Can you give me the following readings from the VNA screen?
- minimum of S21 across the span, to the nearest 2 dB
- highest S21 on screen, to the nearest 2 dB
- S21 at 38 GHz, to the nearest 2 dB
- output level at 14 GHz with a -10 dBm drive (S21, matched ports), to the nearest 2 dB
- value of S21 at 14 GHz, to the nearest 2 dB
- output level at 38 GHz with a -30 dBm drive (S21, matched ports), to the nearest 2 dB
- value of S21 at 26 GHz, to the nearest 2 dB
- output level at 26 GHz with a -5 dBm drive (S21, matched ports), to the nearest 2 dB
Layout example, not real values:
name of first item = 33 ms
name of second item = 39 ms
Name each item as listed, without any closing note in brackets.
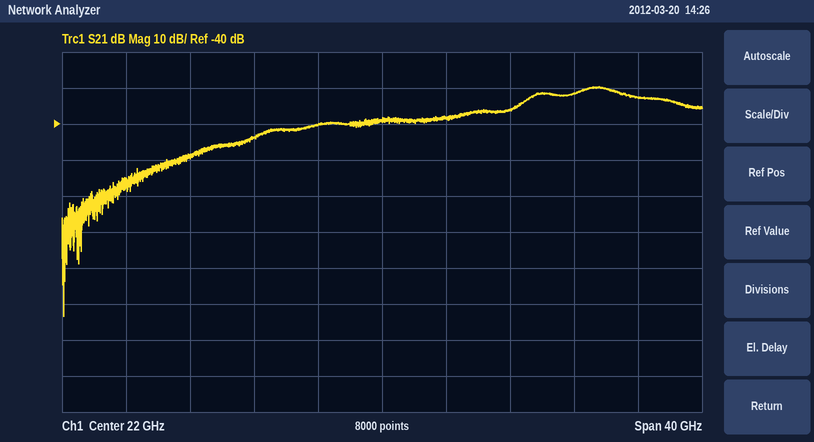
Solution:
minimum of S21 across the span, to the nearest 2 dB = -94 dB
highest S21 on screen, to the nearest 2 dB = -30 dB
S21 at 38 GHz, to the nearest 2 dB = -32 dB
output level at 14 GHz with a -10 dBm drive (S21, matched ports), to the nearest 2 dB = -54 dBm
value of S21 at 14 GHz, to the nearest 2 dB = -44 dB
output level at 38 GHz with a -30 dBm drive (S21, matched ports), to the nearest 2 dB = -62 dBm
value of S21 at 26 GHz, to the nearest 2 dB = -38 dB
output level at 26 GHz with a -5 dBm drive (S21, matched ports), to the nearest 2 dB = -44 dBm
